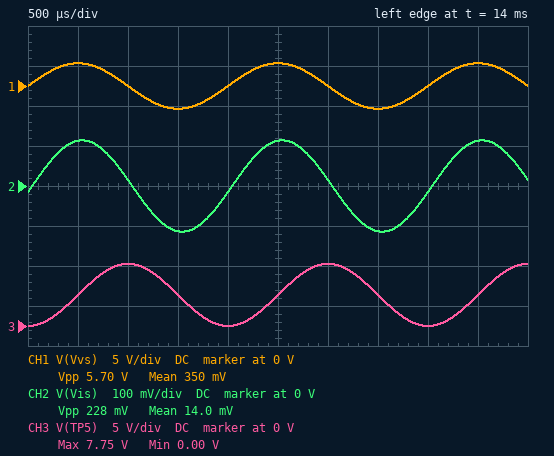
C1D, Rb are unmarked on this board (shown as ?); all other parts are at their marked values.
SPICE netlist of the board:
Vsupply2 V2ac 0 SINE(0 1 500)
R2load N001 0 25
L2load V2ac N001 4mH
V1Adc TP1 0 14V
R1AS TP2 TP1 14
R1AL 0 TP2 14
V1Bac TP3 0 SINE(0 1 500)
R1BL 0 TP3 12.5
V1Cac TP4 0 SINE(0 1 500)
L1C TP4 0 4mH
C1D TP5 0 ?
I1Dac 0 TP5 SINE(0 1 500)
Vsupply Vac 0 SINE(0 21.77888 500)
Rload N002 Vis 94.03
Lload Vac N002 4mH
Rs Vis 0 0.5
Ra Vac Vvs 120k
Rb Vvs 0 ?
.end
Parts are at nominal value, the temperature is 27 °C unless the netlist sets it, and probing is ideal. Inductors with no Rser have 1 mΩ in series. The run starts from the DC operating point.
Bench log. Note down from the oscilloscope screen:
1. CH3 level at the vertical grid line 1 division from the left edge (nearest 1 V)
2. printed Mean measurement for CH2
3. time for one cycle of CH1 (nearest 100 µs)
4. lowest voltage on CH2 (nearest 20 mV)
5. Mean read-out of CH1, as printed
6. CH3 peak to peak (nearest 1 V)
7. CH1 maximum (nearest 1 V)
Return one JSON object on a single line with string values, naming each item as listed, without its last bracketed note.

{"CH3 level at the vertical grid line 1 division from the left edge": "4 V", "printed Mean measurement for CH2": "14.0 mV", "time for one cycle of CH1": "2.0 ms", "lowest voltage on CH2": "-120 mV", "Mean read-out of CH1, as printed": "350 mV", "CH3 peak to peak": "8 V", "CH1 maximum": "3 V"}
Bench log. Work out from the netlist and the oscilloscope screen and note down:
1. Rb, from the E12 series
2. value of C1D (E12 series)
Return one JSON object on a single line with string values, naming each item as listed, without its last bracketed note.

{"Rb, from the E12 series": "18 kΩ", "value of C1D": "82 µF"}
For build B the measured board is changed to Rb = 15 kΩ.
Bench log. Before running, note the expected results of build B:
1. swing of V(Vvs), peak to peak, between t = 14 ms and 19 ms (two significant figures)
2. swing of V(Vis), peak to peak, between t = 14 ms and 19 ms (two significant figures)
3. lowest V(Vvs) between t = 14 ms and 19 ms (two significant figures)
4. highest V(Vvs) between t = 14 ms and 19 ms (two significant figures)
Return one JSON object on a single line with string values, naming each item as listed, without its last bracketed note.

{"swing of V(Vvs), peak to peak, between t = 14 ms and 19 ms": "4.8 V", "swing of V(Vis), peak to peak, between t = 14 ms and 19 ms": "230 mV", "lowest V(Vvs) between t = 14 ms and 19 ms": "-2.4 V", "highest V(Vvs) between t = 14 ms and 19 ms": "2.4 V"}
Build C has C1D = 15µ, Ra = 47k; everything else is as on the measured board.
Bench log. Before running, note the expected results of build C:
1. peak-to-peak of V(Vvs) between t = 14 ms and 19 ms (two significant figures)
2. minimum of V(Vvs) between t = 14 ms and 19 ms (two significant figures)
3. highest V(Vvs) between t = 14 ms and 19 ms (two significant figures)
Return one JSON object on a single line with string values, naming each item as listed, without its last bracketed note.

{"peak-to-peak of V(Vvs) between t = 14 ms and 19 ms": "12 V", "minimum of V(Vvs) between t = 14 ms and 19 ms": "-6.0 V", "highest V(Vvs) between t = 14 ms and 19 ms": "6.0 V"}
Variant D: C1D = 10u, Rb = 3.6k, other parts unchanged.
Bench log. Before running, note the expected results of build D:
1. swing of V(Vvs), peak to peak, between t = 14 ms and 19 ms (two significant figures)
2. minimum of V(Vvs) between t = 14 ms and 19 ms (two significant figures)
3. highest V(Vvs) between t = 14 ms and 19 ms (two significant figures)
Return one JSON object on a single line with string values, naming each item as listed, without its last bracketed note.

{"swing of V(Vvs), peak to peak, between t = 14 ms and 19 ms": "1.3 V", "minimum of V(Vvs) between t = 14 ms and 19 ms": "-630 mV", "highest V(Vvs) between t = 14 ms and 19 ms": "630 mV"}
